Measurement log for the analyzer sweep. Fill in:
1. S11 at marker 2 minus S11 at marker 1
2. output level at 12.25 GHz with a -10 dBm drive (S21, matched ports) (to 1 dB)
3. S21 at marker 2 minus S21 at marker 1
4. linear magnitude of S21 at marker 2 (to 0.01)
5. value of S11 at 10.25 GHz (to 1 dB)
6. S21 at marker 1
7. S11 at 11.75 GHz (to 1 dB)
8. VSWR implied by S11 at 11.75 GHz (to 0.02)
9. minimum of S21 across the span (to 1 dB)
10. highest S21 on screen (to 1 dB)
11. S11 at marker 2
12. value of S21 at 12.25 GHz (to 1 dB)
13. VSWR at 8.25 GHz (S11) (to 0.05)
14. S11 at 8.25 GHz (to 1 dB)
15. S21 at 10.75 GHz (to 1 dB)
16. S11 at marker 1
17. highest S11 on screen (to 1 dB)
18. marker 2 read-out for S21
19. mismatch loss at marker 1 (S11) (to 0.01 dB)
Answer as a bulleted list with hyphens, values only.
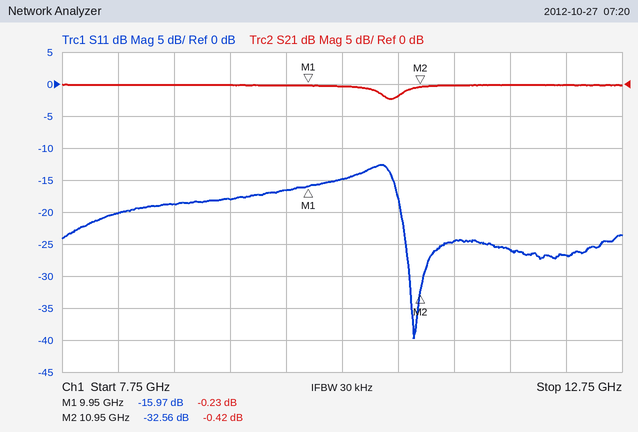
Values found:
- -16.59 dB
- -10 dBm
- -0.19 dB
- 0.95
- -15 dB
- -0.23 dB
- -26 dB
- 1.10
- -2 dB
- 0 dB
- -32.56 dB
- 0 dB
- 1.20
- -20 dB
- -2 dB
- -15.97 dB
- -13 dB
- -0.42 dB
- 0.11 dB
